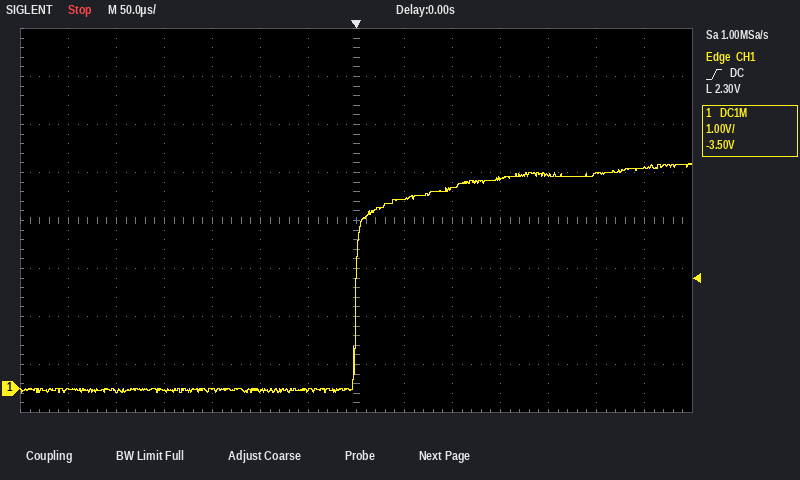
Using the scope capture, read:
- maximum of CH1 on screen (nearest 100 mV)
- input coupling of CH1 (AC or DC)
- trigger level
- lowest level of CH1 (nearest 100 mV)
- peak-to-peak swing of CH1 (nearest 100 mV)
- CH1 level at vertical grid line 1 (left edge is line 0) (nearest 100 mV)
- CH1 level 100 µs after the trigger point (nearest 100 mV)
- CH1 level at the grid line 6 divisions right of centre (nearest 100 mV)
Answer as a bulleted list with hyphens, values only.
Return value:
- 4.7 V
- DC
- 2.30 V
- -100 mV
- 4.8 V
- 0.0 V
- 4.2 V
- 4.6 V
